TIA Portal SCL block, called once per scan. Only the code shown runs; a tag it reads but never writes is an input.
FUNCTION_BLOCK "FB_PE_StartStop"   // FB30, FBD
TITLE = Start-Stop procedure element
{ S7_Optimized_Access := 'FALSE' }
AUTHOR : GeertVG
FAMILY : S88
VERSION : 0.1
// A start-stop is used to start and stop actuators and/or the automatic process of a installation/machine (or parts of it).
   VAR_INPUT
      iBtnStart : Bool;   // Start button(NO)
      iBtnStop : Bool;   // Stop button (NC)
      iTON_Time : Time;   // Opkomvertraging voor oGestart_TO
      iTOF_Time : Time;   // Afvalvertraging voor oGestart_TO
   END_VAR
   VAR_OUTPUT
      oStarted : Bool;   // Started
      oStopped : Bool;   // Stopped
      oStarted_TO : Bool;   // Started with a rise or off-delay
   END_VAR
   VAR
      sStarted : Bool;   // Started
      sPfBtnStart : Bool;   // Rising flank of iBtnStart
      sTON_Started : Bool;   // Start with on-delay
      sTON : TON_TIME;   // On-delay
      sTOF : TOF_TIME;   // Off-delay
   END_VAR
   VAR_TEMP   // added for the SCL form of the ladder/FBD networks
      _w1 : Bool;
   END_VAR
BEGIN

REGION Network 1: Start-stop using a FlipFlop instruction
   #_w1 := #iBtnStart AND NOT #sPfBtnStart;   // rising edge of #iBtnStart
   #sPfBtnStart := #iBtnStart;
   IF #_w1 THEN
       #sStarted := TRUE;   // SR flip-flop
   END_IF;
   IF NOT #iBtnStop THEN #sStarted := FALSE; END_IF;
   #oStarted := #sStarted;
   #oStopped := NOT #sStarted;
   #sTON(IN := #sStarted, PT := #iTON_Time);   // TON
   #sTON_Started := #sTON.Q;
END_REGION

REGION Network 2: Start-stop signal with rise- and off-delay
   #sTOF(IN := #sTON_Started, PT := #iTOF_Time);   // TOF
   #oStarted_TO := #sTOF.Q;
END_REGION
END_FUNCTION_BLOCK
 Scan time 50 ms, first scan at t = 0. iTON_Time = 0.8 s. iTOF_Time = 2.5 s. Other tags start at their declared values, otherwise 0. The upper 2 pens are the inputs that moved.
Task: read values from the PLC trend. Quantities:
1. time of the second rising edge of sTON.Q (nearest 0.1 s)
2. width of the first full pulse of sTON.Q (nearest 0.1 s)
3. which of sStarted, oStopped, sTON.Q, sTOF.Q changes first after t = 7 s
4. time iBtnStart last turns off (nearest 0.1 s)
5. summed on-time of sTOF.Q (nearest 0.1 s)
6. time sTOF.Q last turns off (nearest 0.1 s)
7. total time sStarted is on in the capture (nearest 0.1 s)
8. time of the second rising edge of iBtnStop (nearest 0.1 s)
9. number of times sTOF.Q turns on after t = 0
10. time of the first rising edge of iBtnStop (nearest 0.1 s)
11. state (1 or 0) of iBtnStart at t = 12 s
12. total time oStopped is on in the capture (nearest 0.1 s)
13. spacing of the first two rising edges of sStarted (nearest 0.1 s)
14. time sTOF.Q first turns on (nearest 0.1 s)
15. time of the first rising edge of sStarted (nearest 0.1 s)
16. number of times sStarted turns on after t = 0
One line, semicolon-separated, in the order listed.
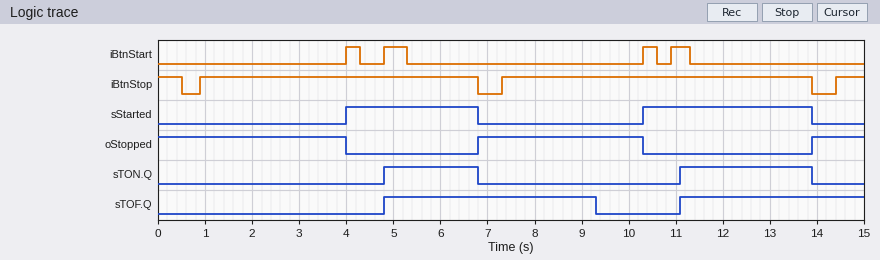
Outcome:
11.1 s; 2.0 s; sTOF.Q; 11.3 s; 8.4 s; 9.3 s; 6.4 s; 7.3 s; 2; 0.9 s; 0; 8.6 s; 6.3 s; 4.8 s; 4.0 s; 2
